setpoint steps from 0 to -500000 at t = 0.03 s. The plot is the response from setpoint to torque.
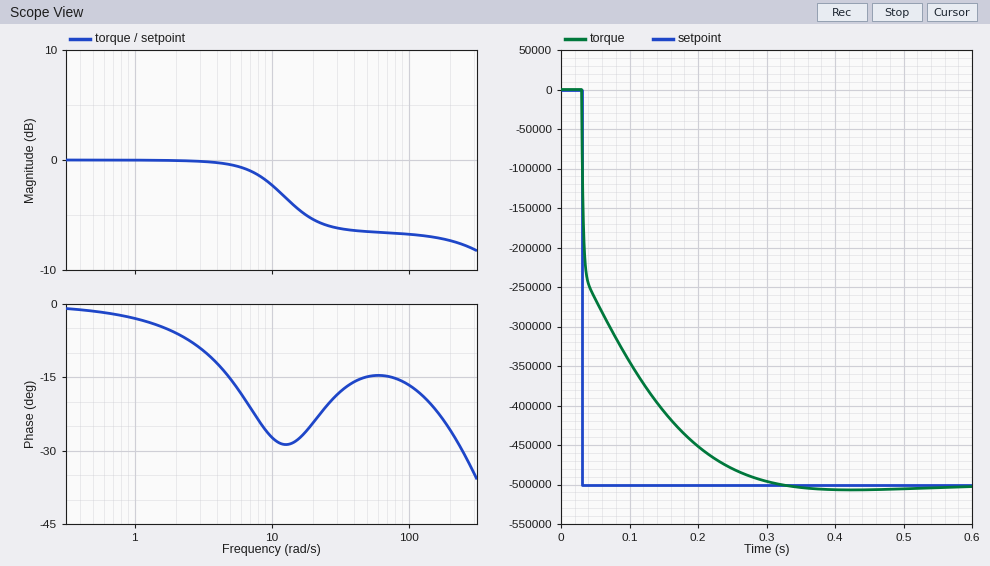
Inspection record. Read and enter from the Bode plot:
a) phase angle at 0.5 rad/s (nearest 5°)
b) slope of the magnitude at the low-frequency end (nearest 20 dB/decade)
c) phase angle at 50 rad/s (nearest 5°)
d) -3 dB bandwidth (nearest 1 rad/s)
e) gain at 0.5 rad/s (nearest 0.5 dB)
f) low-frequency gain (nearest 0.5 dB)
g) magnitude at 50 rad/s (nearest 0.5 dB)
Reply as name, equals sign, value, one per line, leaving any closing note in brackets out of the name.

phase angle at 0.5 rad/s = 0°
slope of the magnitude at the low-frequency end = 0 dB/decade
phase angle at 50 rad/s = -15°
-3 dB bandwidth = 12 rad/s
gain at 0.5 rad/s = 0.0 dB
low-frequency gain = 0.0 dB
magnitude at 50 rad/s = -6.5 dB
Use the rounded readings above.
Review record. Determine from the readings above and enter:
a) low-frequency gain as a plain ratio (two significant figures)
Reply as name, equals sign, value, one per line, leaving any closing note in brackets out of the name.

low-frequency gain as a plain ratio = 1.0
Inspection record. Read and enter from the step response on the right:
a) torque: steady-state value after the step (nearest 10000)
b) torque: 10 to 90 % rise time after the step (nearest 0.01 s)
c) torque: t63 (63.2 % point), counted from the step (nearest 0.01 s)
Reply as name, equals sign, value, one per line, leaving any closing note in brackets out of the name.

torque: steady-state value after the step = -500000
torque: 10 to 90 % rise time after the step = 0.17 s
torque: t63 (63.2 % point), counted from the step = 0.05 s
